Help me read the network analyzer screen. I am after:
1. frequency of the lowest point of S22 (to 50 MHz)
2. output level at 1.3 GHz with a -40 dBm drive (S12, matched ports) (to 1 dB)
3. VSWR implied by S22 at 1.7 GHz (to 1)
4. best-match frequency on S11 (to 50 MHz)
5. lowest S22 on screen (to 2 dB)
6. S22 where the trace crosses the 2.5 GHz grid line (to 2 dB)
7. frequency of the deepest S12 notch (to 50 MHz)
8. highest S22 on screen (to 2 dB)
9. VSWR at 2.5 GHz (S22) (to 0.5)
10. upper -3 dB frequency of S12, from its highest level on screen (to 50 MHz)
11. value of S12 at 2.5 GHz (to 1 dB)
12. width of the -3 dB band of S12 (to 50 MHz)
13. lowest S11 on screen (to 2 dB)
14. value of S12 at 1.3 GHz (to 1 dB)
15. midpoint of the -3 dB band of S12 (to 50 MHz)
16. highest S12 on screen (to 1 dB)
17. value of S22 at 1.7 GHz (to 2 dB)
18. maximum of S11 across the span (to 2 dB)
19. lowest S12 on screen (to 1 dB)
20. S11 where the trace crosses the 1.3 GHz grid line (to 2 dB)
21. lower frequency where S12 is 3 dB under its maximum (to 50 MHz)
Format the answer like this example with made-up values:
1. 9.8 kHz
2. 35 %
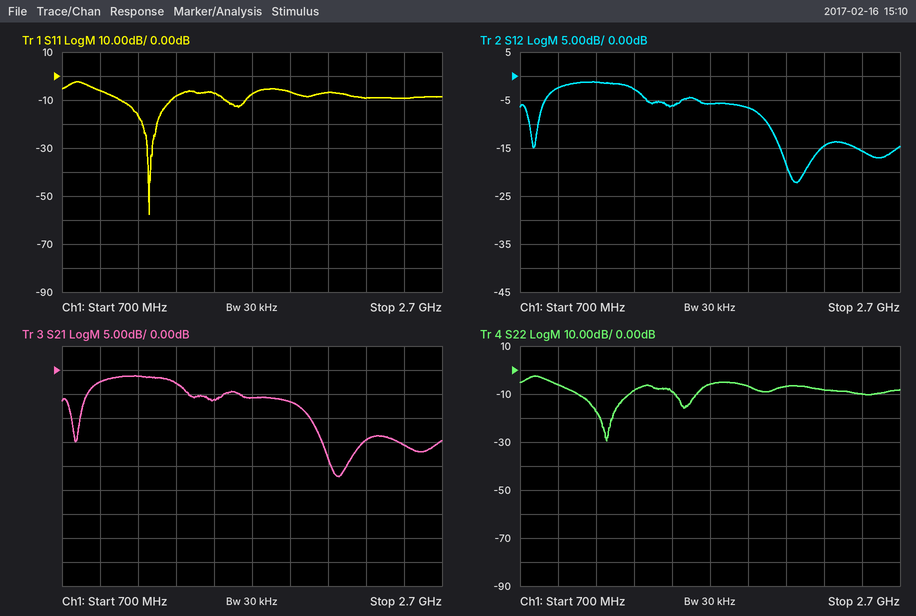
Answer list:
1. 1.15 GHz
2. -43 dBm
3. 3
4. 1.15 GHz
5. -30 dB
6. -10 dB
7. 2.15 GHz
8. -2 dB
9. 2.0
10. 1.35 GHz
11. -16 dB
12. 500 MHz
13. -58 dB
14. -3 dB
15. 1.10 GHz
16. -1 dB
17. -6 dB
18. -2 dB
19. -22 dB
20. -8 dB
21. 850 MHz
